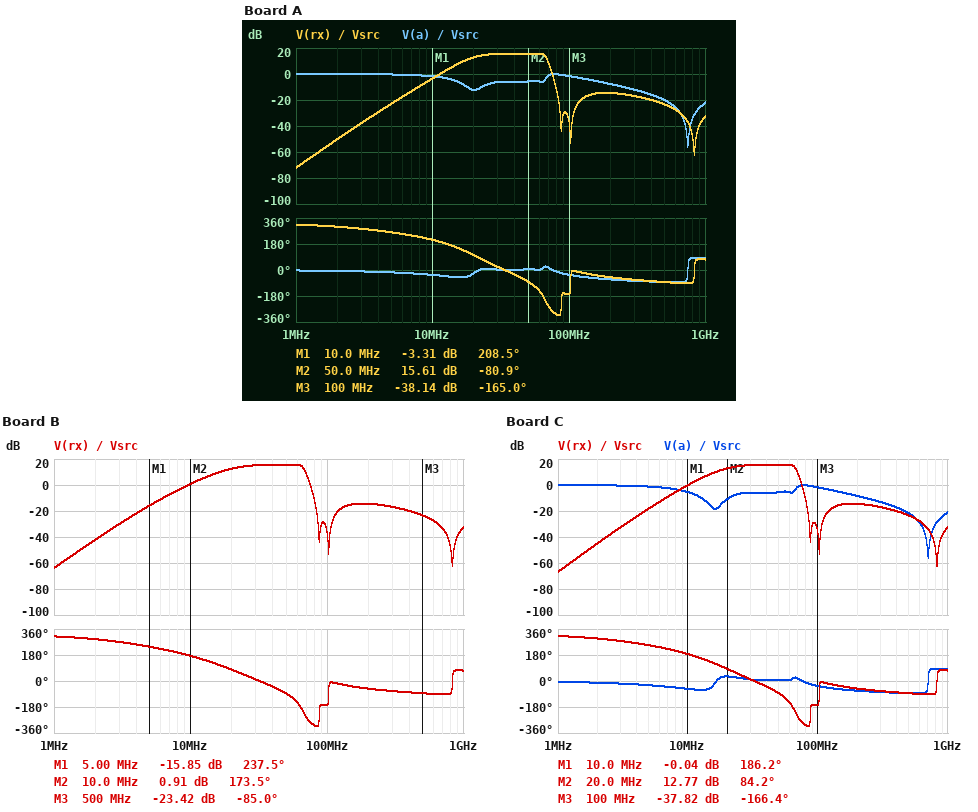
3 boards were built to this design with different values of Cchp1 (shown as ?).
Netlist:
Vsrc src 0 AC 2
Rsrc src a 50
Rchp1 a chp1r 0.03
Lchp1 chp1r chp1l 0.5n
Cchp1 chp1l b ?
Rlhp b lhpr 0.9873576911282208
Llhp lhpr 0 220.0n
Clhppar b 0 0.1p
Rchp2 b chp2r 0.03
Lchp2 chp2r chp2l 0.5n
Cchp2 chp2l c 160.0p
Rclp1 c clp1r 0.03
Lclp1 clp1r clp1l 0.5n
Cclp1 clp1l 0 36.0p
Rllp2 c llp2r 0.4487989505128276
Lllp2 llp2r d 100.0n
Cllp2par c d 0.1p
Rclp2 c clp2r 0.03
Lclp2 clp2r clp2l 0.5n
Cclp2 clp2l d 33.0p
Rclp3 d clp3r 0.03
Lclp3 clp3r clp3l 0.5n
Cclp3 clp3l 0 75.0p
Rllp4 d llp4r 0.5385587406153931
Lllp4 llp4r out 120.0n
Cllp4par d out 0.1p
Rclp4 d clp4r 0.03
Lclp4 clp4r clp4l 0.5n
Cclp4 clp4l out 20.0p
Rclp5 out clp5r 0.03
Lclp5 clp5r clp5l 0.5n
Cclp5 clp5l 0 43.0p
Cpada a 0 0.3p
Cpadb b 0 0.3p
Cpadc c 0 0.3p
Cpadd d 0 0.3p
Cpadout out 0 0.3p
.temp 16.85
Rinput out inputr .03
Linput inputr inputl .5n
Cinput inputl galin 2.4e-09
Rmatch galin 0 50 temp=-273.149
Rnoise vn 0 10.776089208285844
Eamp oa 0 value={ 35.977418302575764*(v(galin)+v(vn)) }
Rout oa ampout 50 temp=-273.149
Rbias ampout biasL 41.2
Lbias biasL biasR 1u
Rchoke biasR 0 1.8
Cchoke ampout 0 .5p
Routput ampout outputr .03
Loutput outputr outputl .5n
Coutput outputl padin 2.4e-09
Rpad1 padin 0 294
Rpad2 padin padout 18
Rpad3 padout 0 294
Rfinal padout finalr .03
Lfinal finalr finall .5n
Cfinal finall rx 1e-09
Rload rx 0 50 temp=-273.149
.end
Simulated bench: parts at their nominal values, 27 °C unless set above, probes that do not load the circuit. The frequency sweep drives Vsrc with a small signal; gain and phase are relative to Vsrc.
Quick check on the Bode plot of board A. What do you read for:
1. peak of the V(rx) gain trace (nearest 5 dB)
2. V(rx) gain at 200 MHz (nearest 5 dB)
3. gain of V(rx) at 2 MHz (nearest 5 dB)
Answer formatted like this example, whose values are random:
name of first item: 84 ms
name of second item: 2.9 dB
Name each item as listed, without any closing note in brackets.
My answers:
peak of the V(rx) gain trace: 15 dB
V(rx) gain at 200 MHz: -15 dB
gain of V(rx) at 2 MHz: -50 dB
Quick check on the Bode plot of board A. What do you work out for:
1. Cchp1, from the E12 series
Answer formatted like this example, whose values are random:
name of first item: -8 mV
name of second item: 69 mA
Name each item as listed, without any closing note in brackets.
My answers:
Cchp1, from the E12 series: 180 pF
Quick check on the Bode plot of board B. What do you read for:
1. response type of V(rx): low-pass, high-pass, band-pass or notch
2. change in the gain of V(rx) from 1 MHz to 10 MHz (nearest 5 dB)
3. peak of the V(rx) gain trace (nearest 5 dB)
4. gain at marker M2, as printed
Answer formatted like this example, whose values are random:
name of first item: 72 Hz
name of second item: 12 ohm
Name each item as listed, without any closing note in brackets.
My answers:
response type of V(rx): low-pass, high-pass, band-pass or notch: band-pass
change in the gain of V(rx) from 1 MHz to 10 MHz: 65 dB
peak of the V(rx) gain trace: 15 dB
gain at marker M2, as printed: 0.91 dB
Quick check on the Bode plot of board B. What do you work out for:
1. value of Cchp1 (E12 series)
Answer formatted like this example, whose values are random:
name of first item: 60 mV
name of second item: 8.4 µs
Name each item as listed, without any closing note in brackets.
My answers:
value of Cchp1: 470 pF
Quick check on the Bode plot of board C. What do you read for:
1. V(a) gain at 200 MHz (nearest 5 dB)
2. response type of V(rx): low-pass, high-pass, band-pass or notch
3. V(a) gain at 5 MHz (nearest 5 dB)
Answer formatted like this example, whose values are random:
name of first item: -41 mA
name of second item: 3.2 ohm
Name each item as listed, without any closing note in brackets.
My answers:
V(a) gain at 200 MHz: -10 dB
response type of V(rx): low-pass, high-pass, band-pass or notch: band-pass
V(a) gain at 5 MHz: 0 dB
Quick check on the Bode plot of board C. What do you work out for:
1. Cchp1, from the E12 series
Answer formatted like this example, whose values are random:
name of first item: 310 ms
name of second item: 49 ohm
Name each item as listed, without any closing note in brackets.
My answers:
Cchp1, from the E12 series: 330 pF
